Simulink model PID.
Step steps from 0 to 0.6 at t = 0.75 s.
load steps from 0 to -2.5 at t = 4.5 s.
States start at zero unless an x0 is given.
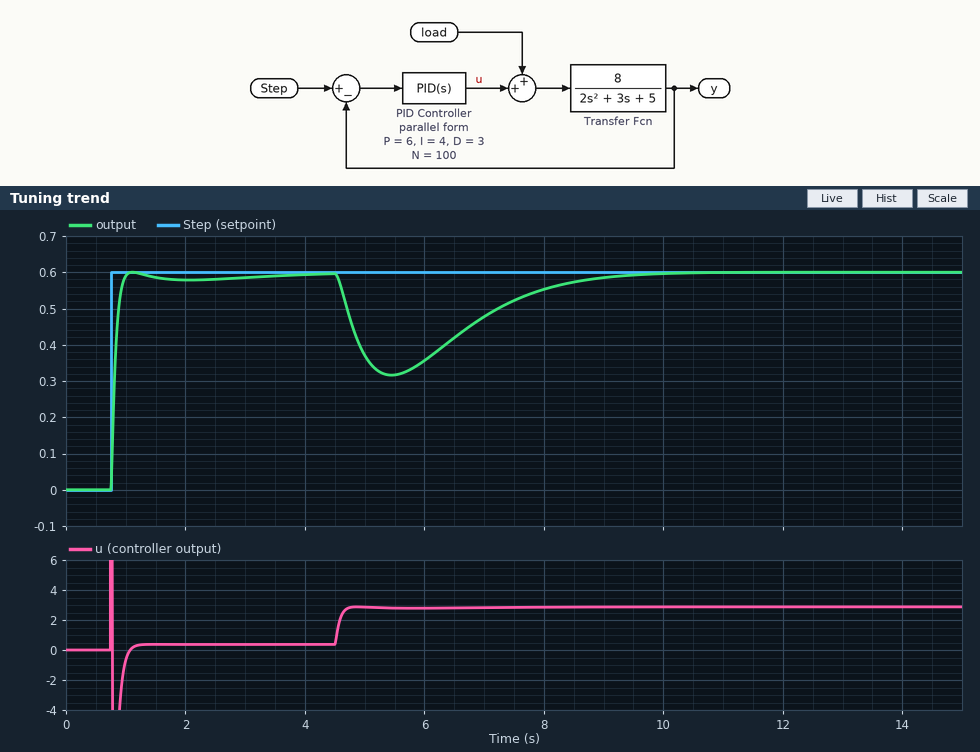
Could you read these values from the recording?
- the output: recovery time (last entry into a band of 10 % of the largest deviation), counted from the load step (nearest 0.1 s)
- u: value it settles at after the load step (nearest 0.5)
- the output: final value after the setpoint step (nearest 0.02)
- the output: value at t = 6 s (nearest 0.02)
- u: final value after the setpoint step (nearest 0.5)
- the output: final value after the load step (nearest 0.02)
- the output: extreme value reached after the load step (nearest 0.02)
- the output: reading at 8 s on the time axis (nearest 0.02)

4.0 s
3.0
0.60
0.36
0.5
0.60
0.32
0.56
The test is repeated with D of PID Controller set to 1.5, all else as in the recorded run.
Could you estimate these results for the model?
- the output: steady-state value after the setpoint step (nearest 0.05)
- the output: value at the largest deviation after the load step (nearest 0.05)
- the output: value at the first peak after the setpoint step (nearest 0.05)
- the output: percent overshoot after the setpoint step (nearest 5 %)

0.60
0.25
0.65
10 %
